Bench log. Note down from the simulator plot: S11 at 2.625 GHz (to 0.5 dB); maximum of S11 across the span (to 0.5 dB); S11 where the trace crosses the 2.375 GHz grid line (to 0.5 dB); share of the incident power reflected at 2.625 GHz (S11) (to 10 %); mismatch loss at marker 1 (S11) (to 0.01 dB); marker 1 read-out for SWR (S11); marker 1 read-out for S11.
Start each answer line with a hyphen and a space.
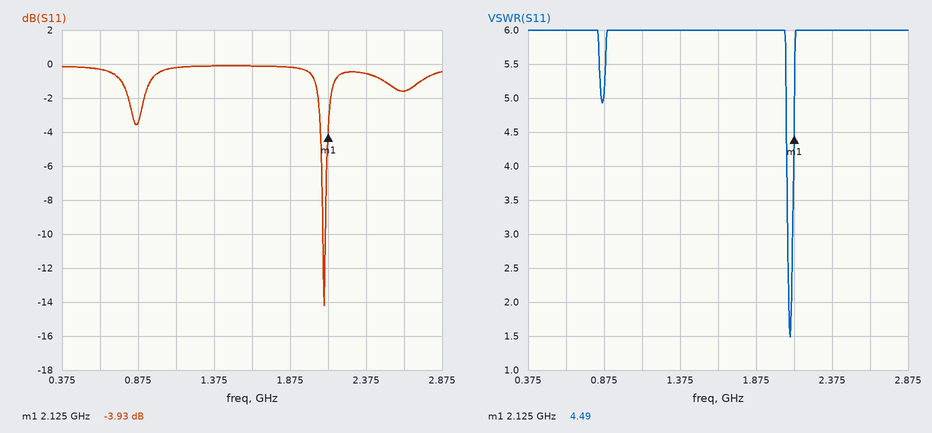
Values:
- -1.5 dB
- 0.0 dB
- -0.5 dB
- 70 %
- 2.25 dB
- 4.49
- -3.93 dB
